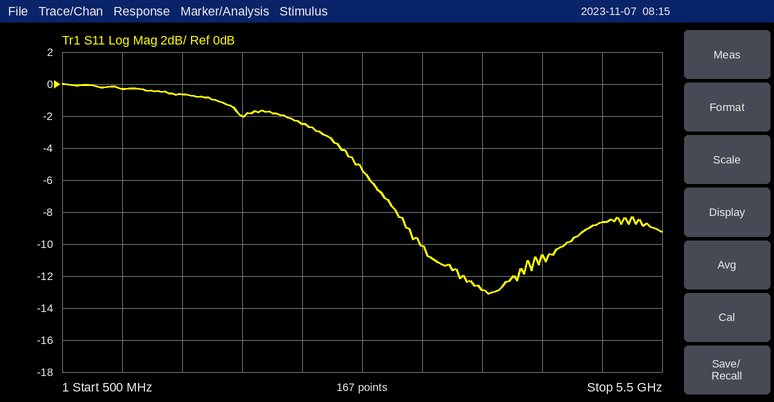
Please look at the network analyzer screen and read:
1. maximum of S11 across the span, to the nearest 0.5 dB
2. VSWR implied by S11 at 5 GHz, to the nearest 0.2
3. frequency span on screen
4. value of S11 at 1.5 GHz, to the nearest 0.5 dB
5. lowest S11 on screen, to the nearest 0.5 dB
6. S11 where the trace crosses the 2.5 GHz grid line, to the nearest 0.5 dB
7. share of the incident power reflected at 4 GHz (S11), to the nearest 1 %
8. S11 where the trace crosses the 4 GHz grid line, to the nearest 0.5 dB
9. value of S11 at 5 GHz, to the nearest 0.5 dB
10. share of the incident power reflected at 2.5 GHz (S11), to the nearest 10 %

0.0 dB
2.2
5 GHz
-0.5 dB
-13.0 dB
-2.5 dB
5 %
-13.0 dB
-8.5 dB
60 %
